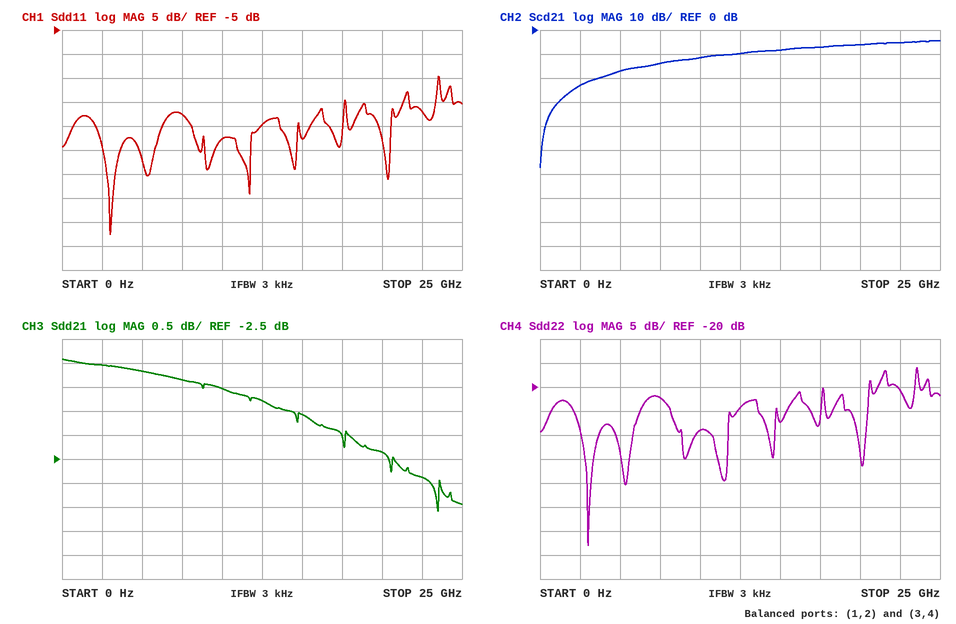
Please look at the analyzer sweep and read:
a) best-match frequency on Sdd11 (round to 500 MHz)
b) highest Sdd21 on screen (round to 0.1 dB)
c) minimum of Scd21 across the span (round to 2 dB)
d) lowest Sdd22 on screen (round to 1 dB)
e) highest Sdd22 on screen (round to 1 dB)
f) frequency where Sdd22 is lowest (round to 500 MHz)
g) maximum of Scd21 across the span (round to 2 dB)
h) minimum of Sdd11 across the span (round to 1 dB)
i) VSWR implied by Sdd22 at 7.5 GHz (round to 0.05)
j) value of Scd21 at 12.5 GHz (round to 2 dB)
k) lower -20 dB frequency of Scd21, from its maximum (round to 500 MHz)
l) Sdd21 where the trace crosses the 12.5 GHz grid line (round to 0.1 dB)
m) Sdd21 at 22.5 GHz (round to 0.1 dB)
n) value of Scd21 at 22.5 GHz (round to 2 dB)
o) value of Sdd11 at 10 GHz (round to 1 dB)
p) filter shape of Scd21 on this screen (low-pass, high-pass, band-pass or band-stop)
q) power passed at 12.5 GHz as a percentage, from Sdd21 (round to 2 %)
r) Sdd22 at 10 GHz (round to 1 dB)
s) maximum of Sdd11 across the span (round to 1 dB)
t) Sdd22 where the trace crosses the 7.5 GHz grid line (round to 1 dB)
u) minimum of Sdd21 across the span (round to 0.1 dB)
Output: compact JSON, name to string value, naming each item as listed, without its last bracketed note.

{"best-match frequency on Sdd11": "3.0 GHz", "highest Sdd21 on screen": "-0.4 dB", "minimum of Scd21 across the span": "-58 dB", "lowest Sdd22 on screen": "-53 dB", "highest Sdd22 on screen": "-16 dB", "frequency where Sdd22 is lowest": "3.0 GHz", "maximum of Scd21 across the span": "-4 dB", "minimum of Sdd11 across the span": "-48 dB", "VSWR implied by Sdd22 at 7.5 GHz": "1.15", "value of Scd21 at 12.5 GHz": "-10 dB", "lower -20 dB frequency of Scd21, from its maximum": "2.0 GHz", "Sdd21 where the trace crosses the 12.5 GHz grid line": "-1.3 dB", "Sdd21 at 22.5 GHz": "-2.9 dB", "value of Scd21 at 22.5 GHz": "-6 dB", "value of Sdd11 at 10 GHz": "-28 dB", "filter shape of Scd21 on this screen": "high-pass", "power passed at 12.5 GHz as a percentage, from Sdd21": "74 %", "Sdd22 at 10 GHz": "-29 dB", "maximum of Sdd11 across the span": "-15 dB", "Sdd22 where the trace crosses the 7.5 GHz grid line": "-22 dB", "minimum of Sdd21 across the span": "-3.6 dB"}
